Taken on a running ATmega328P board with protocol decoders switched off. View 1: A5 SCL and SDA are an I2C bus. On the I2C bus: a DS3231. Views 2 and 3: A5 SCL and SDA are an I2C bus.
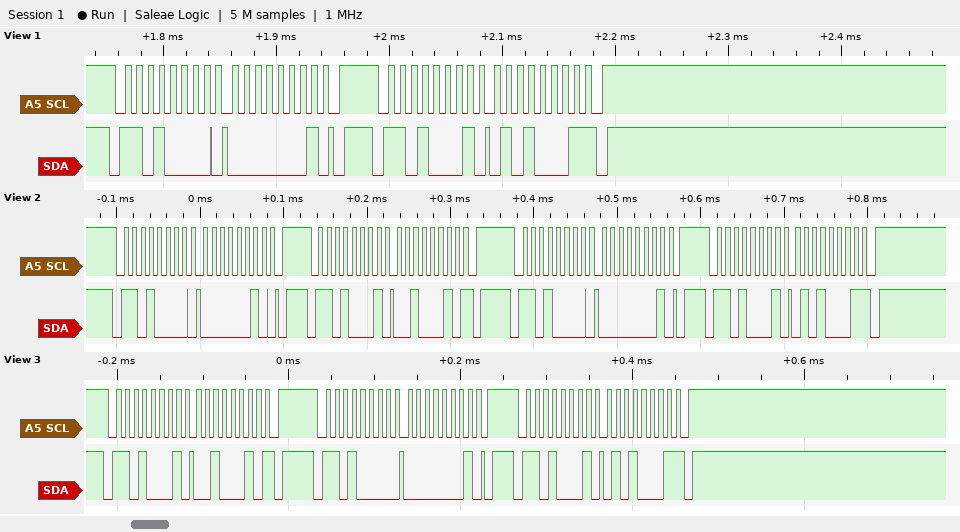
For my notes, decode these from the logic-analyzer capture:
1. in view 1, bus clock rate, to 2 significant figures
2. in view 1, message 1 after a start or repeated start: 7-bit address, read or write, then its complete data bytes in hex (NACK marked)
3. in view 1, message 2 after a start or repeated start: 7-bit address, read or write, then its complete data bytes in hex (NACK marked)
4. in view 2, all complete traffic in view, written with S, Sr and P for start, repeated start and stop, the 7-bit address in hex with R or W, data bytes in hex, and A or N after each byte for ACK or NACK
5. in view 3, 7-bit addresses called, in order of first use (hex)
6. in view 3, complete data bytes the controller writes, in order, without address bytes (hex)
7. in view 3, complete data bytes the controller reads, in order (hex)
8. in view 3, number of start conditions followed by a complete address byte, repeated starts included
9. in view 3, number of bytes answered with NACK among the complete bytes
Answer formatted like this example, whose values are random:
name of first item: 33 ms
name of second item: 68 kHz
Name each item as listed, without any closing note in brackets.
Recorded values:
in view 1, bus clock rate, to 2 significant figures: 100 kHz
in view 1, message 1 after a start or repeated start: 7-bit address, read or write, then its complete data bytes in hex: 0x68 write: 01
in view 1, message 2 after a start or repeated start: 7-bit address, read or write, then its complete data bytes in hex: 0x68 read: 51 NACK
in view 2, all complete traffic in view, written with S, Sr and P for start, repeated start and stop, the 7-bit address in hex with R or W, data bytes in hex, and A or N after each byte for ACK or NACK: S 68W A 02 A P S 68R A 22 N P S 68W A 01 A P S 68R A 51 N P
in view 3, 7-bit addresses called, in order of first use: 0x68
in view 3, complete data bytes the controller writes, in order, without address bytes: 01
in view 3, complete data bytes the controller reads, in order: 22 51
in view 3, number of start conditions followed by a complete address byte, repeated starts included: 3
in view 3, number of bytes answered with NACK among the complete bytes: 2
